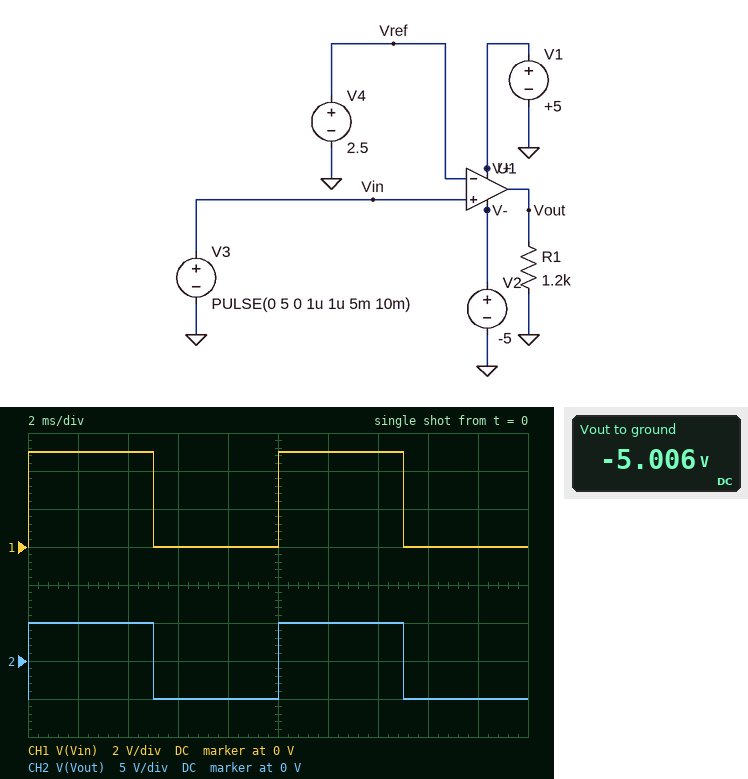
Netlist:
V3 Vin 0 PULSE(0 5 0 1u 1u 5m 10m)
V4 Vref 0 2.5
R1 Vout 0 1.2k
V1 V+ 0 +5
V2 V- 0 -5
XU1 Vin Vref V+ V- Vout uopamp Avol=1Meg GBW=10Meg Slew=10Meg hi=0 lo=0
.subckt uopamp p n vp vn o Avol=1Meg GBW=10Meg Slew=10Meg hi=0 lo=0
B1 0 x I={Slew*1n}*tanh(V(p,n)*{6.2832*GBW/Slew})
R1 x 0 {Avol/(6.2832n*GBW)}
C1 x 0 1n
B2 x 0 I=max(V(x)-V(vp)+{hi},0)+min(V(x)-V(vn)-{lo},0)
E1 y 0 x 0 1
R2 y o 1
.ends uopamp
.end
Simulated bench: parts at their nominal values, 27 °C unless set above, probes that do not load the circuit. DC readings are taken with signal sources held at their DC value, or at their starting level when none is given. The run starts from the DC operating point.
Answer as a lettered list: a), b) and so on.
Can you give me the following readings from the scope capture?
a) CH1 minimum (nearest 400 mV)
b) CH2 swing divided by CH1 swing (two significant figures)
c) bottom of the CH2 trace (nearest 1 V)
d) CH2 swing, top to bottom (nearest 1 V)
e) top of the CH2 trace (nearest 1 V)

a) 0 V
b) 2.0
c) -5 V
d) 10 V
e) 5 V
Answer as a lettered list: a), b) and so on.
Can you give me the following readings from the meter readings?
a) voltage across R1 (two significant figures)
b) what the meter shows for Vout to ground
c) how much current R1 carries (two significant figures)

a) 5.0 V
b) -5.006 V
c) 4.2 mA
